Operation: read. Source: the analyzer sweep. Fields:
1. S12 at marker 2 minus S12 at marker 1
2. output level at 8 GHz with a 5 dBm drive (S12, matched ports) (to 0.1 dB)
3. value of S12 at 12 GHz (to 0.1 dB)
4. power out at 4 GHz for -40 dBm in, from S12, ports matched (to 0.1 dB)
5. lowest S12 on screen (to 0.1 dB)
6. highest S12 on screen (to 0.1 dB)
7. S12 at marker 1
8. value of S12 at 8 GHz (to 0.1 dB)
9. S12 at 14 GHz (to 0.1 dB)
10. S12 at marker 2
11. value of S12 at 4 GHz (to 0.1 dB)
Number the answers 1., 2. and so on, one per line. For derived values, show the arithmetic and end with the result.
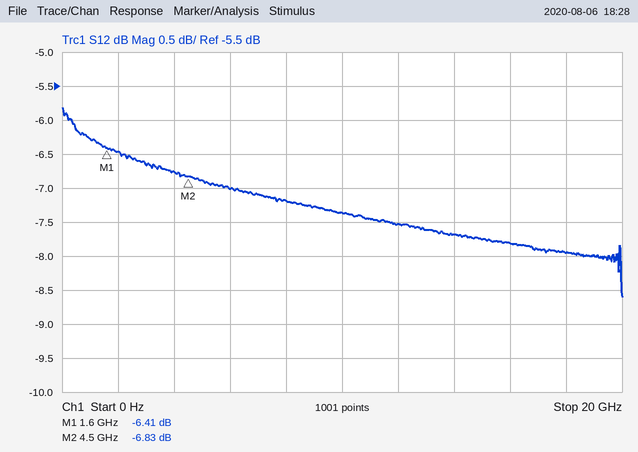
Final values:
1. -6.83 − (-6.41) = -0.42 dB
2. 5 dBm + (-7.2 dB) = -2.2 dBm
3. -7.5 dB
4. -40 dBm + (-6.8 dB) = -46.8 dBm
5. -8.6 dB
6. -5.8 dB
7. -6.41 dB
8. -7.2 dB
9. -7.7 dB
10. -6.83 dB
11. -6.8 dB
